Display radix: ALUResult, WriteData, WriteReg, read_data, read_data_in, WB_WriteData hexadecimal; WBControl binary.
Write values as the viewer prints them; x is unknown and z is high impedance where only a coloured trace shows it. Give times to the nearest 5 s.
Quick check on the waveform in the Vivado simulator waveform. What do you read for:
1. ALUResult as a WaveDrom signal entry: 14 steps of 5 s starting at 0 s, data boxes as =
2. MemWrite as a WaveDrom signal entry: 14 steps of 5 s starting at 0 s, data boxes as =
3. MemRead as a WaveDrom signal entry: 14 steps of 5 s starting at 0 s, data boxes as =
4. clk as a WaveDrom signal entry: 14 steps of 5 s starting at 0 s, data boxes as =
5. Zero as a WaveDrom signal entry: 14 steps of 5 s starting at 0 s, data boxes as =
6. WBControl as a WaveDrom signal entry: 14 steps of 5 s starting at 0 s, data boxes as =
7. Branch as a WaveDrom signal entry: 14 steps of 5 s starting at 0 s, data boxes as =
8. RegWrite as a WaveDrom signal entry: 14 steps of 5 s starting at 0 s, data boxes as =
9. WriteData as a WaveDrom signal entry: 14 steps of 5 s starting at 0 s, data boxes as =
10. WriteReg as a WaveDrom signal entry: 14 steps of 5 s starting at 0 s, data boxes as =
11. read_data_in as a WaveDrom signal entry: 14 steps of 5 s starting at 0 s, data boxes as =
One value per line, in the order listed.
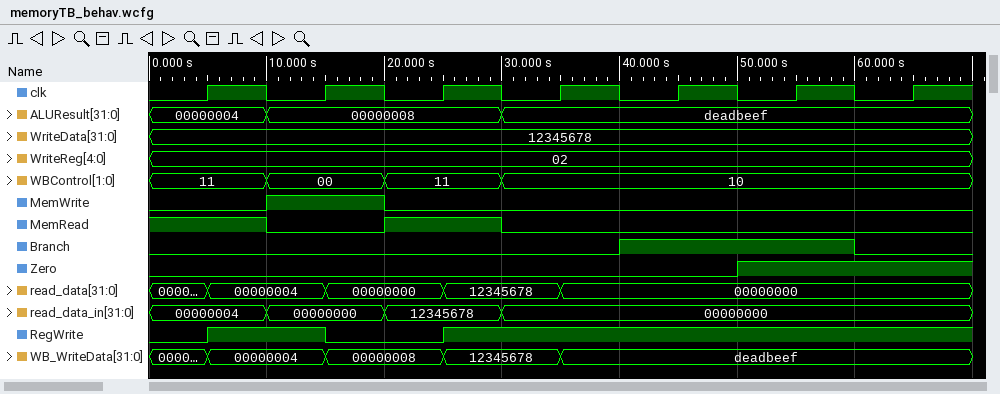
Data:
{name: 'ALUResult', wave: '=.=...=.......', data: '00000004 00000008 deadbeef'}
{name: 'MemWrite', wave: '0.1.0.........'}
{name: 'MemRead', wave: '1.0.1.0.......'}
{name: 'clk', wave: '01010101010101'}
{name: 'Zero', wave: '0.........1...'}
{name: 'WBControl', wave: '=.=.=.=.......', data: '11 00 11 10'}
{name: 'Branch', wave: '0.......1...0.'}
{name: 'RegWrite', wave: '01.0.1........'}
{name: 'WriteData', wave: '=.............', data: '12345678'}
{name: 'WriteReg', wave: '=.............', data: '02'}
{name: 'read_data_in', wave: '=.=.=.=.......', data: '00000004 00000000 12345678 00000000'}
